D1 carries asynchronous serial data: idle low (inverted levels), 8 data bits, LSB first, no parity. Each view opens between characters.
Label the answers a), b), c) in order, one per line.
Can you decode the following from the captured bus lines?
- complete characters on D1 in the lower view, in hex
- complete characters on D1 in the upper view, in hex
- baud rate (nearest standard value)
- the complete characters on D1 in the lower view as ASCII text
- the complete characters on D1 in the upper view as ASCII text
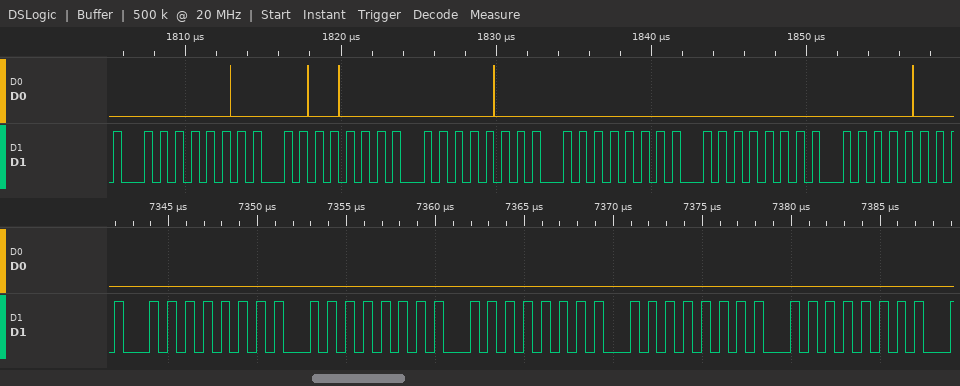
a) 57, 55, 55, 75, 55, 5D, 55, 57, 55
b) 57, 55, 55, 75, 55, 5D, 55, 57, 55, 55
c) 2000000 baud
d) "WUUuU]UWU"
e) "WUUuU]UWUU"
